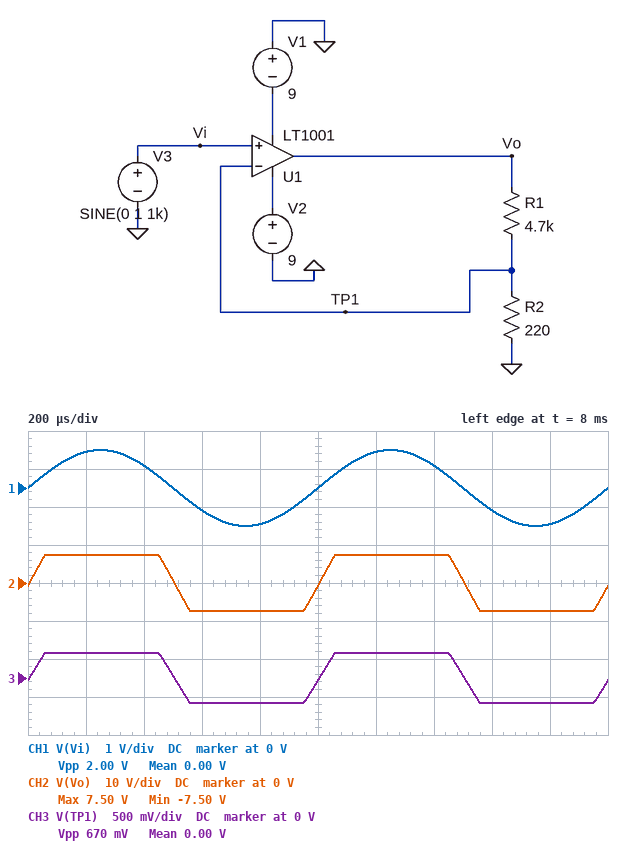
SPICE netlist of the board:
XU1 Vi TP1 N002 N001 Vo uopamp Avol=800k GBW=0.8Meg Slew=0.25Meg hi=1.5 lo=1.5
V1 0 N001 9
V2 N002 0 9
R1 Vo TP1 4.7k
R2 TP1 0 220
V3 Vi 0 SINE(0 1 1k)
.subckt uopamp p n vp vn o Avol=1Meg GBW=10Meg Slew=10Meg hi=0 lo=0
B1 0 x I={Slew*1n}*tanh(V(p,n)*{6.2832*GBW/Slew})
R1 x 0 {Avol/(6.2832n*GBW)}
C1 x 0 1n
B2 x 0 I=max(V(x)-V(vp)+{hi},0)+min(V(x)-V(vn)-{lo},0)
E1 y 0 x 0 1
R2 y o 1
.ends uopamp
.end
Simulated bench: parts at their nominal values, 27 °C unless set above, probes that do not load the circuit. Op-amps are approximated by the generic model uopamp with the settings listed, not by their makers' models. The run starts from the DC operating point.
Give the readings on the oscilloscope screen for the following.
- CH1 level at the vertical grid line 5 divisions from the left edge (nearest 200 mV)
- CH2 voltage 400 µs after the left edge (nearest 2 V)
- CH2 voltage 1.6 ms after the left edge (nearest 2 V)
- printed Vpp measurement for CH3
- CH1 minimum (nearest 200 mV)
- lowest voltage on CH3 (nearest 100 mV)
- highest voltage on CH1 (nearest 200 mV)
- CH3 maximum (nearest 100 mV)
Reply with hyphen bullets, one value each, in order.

- 0 V
- 8 V
- -8 V
- 670 mV
- -1.0 V
- -300 mV
- 1.0 V
- 300 mV
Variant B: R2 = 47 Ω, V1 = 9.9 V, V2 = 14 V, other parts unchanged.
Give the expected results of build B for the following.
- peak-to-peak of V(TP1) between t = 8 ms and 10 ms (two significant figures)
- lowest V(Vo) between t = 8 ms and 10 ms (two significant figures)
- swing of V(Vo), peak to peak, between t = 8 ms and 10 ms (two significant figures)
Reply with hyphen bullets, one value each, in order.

- 210 mV
- -8.4 V
- 21 V
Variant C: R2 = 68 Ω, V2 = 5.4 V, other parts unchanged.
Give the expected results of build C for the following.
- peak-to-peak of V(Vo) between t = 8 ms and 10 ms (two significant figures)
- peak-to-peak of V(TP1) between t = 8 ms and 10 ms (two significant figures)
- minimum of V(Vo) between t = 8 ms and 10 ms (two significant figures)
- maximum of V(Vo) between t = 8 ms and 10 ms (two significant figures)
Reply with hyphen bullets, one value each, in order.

- 11 V
- 160 mV
- -7.5 V
- 3.9 V
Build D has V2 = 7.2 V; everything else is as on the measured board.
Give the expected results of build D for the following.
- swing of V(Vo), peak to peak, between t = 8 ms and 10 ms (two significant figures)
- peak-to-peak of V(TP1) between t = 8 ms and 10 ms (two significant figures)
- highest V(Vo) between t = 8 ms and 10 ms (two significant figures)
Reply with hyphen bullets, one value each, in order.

- 13 V
- 590 mV
- 5.7 V
